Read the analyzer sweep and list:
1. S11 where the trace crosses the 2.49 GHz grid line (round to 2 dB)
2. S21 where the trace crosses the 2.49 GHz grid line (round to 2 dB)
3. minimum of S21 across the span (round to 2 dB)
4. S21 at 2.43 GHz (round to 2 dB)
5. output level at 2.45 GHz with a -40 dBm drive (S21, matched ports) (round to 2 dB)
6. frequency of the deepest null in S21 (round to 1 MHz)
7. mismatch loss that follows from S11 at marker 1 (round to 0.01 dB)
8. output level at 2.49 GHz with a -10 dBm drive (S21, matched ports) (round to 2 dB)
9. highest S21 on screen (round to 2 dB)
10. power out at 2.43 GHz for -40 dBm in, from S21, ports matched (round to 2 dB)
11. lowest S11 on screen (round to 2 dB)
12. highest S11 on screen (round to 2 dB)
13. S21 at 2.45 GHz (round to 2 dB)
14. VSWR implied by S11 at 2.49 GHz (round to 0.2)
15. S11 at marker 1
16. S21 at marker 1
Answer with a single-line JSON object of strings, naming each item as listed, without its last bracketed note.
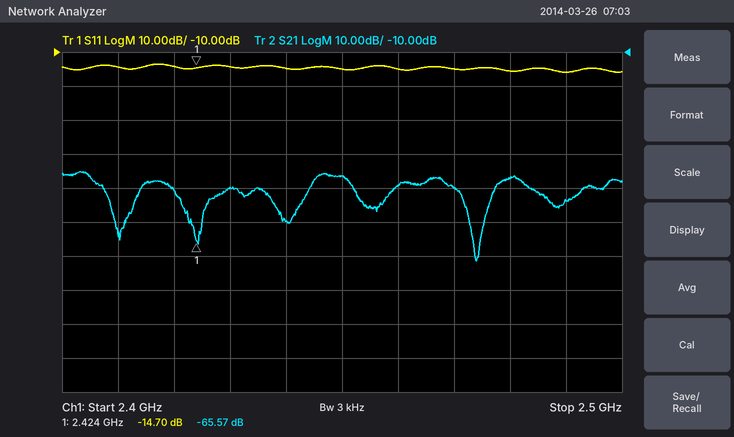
{"S11 where the trace crosses the 2.49 GHz grid line": "-16 dB", "S21 where the trace crosses the 2.49 GHz grid line": "-54 dB", "minimum of S21 across the span": "-72 dB", "S21 at 2.43 GHz": "-50 dB", "output level at 2.45 GHz with a -40 dBm drive (S21, matched ports)": "-86 dBm", "frequency of the deepest null in S21": "2.474 GHz", "mismatch loss that follows from S11 at marker 1": "0.15 dB", "output level at 2.49 GHz with a -10 dBm drive (S21, matched ports)": "-64 dBm", "highest S21 on screen": "-46 dB", "power out at 2.43 GHz for -40 dBm in, from S21, ports matched": "-90 dBm", "lowest S11 on screen": "-16 dB", "highest S11 on screen": "-14 dB", "S21 at 2.45 GHz": "-46 dB", "VSWR implied by S11 at 2.49 GHz": "1.4", "S11 at marker 1": "-14.70 dB", "S21 at marker 1": "-65.57 dB"}
